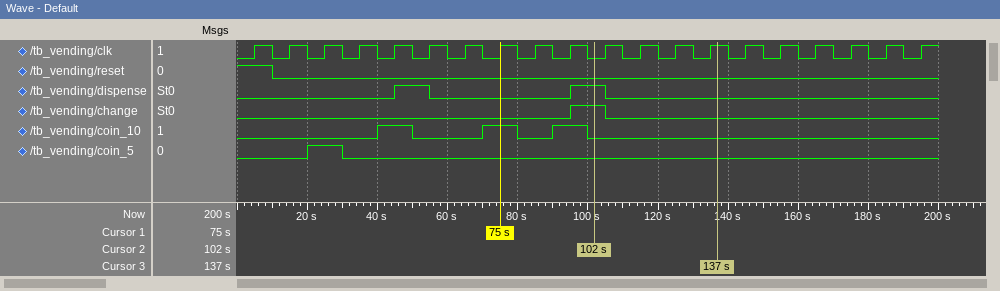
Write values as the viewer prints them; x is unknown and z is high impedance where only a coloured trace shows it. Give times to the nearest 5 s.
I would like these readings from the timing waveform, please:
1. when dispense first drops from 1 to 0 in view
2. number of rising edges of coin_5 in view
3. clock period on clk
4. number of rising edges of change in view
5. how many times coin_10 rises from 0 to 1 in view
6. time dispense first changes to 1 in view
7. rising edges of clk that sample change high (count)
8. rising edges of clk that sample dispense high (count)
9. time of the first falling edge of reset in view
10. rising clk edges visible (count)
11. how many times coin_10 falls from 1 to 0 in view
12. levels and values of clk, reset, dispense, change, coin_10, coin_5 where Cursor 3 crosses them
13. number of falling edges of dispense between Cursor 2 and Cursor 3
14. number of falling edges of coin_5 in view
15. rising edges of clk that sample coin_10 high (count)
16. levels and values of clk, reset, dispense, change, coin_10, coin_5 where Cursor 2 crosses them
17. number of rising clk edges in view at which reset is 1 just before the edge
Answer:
55 s
1
10 s
1
3
45 s
1
2
10 s
20
3
clk=1, reset=0, dispense=0, change=0, coin_10=0, coin_5=0
1
1
3
clk=0, reset=0, dispense=1, change=1, coin_10=0, coin_5=0
1
